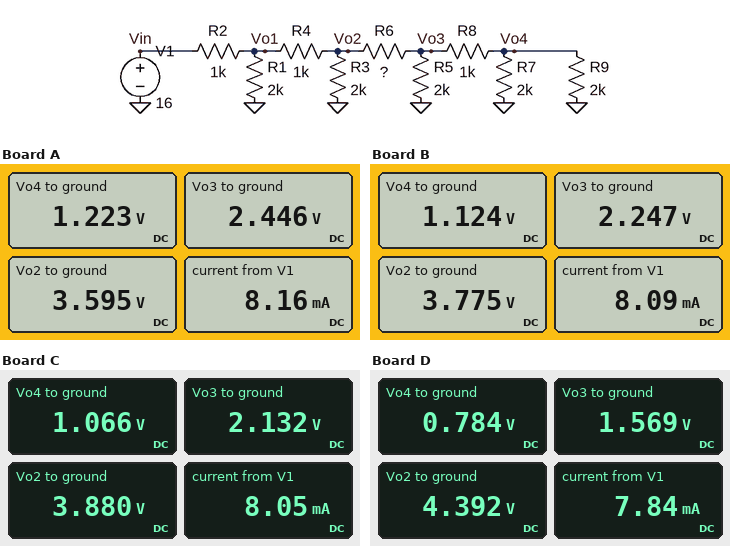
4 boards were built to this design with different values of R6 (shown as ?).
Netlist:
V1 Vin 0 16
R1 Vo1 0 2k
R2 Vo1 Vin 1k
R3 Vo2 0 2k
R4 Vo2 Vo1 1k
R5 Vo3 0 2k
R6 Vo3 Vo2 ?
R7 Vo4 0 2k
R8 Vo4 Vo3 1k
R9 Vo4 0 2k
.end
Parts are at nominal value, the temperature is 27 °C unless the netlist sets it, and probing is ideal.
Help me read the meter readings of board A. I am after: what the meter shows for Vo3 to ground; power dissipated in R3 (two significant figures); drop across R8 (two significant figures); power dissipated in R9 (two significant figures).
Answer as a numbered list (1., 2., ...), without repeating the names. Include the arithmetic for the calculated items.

1. 2.446 V
2. (3.595 V)^2 / 2 kΩ = 6.5 mW
3. 2.446 V - 1.223 V = 1.2 V
4. (1.223 V)^2 / 2 kΩ = 750 µW
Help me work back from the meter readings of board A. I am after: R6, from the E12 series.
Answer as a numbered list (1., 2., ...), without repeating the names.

1. 470 Ω
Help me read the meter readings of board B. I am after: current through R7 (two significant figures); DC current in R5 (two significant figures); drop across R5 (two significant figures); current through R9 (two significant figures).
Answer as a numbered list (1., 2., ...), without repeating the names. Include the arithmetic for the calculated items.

1. (1.124 V) / 2 kΩ = 560 µA
2. (2.247 V) / 2 kΩ = 1.1 mA
3. 2.247 V = 2.2 V
4. (1.124 V) / 2 kΩ = 560 µA
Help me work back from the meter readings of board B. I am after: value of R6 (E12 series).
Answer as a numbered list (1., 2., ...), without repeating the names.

1. 680 Ω
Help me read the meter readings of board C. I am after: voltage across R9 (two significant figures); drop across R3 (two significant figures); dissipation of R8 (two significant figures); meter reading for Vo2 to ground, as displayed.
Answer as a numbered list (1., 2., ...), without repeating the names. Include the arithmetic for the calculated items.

1. 1.066 V = 1.1 V
2. 3.88 V = 3.9 V
3. (2.132 V - 1.066 V)^2 / 1 kΩ = 1.1 mW
4. 3.880 V
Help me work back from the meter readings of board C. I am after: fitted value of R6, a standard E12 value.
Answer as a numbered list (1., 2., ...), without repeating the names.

1. 820 Ω
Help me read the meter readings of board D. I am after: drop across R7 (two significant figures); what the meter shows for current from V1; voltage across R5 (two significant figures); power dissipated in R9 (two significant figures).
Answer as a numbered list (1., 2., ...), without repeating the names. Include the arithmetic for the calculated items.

1. 784 mV = 780 mV
2. 7.84 mA
3. 1.569 V = 1.6 V
4. (784 mV)^2 / 2 kΩ = 310 µW
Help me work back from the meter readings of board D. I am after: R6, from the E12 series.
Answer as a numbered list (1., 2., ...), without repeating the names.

1. 1.8 kΩ
